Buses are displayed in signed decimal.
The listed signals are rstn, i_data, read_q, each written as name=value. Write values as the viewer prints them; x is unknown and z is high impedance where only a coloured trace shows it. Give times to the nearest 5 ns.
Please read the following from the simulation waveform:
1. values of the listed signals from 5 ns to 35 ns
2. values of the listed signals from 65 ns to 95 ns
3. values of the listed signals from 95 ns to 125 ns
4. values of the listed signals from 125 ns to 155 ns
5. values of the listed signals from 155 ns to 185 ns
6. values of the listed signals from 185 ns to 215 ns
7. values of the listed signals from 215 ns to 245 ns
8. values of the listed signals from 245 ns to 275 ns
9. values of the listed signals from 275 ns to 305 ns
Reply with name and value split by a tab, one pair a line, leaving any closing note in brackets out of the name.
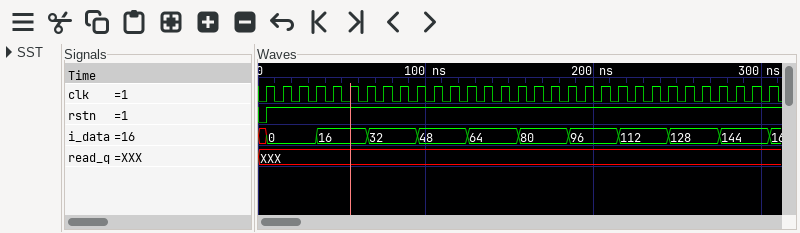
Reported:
values of the listed signals from 5 ns to 35 ns	rstn=1, i_data=0, read_q=XXX
values of the listed signals from 65 ns to 95 ns	rstn=1, i_data=32, read_q=XXX
values of the listed signals from 95 ns to 125 ns	rstn=1, i_data=48, read_q=XXX
values of the listed signals from 125 ns to 155 ns	rstn=1, i_data=64, read_q=XXX
values of the listed signals from 155 ns to 185 ns	rstn=1, i_data=80, read_q=XXX
values of the listed signals from 185 ns to 215 ns	rstn=1, i_data=96, read_q=XXX
values of the listed signals from 215 ns to 245 ns	rstn=1, i_data=112, read_q=XXX
values of the listed signals from 245 ns to 275 ns	rstn=1, i_data=128, read_q=XXX
values of the listed signals from 275 ns to 305 ns	rstn=1, i_data=144, read_q=XXX
